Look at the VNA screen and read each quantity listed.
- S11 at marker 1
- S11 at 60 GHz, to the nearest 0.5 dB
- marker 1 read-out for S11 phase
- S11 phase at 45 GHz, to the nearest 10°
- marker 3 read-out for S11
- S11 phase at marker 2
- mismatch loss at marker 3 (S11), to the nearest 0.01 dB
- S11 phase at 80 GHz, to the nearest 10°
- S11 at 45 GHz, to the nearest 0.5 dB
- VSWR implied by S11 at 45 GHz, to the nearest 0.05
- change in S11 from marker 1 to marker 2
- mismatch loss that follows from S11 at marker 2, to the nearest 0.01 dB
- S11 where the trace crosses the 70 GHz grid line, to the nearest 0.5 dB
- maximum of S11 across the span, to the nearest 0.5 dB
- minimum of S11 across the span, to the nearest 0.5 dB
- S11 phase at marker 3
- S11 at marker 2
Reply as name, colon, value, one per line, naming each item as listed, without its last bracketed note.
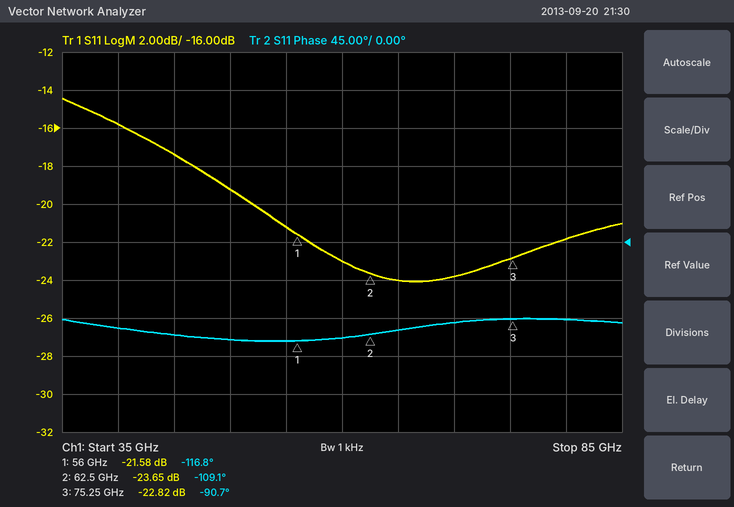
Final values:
S11 at marker 1: -21.58 dB
S11 at 60 GHz, to the nearest 0.5 dB: -23.0 dB
marker 1 read-out for S11 phase: -116.8°
S11 phase at 45 GHz, to the nearest 10°: -110°
marker 3 read-out for S11: -22.82 dB
S11 phase at marker 2: -109.1°
mismatch loss at marker 3 (S11), to the nearest 0.01 dB: 0.02 dB
S11 phase at 80 GHz, to the nearest 10°: -90°
S11 at 45 GHz, to the nearest 0.5 dB: -17.5 dB
VSWR implied by S11 at 45 GHz, to the nearest 0.05: 1.30
change in S11 from marker 1 to marker 2: -2.07 dB
mismatch loss that follows from S11 at marker 2, to the nearest 0.01 dB: 0.02 dB
S11 where the trace crosses the 70 GHz grid line, to the nearest 0.5 dB: -24.0 dB
maximum of S11 across the span, to the nearest 0.5 dB: -14.5 dB
minimum of S11 across the span, to the nearest 0.5 dB: -24.0 dB
S11 phase at marker 3: -90.7°
S11 at marker 2: -23.65 dB
